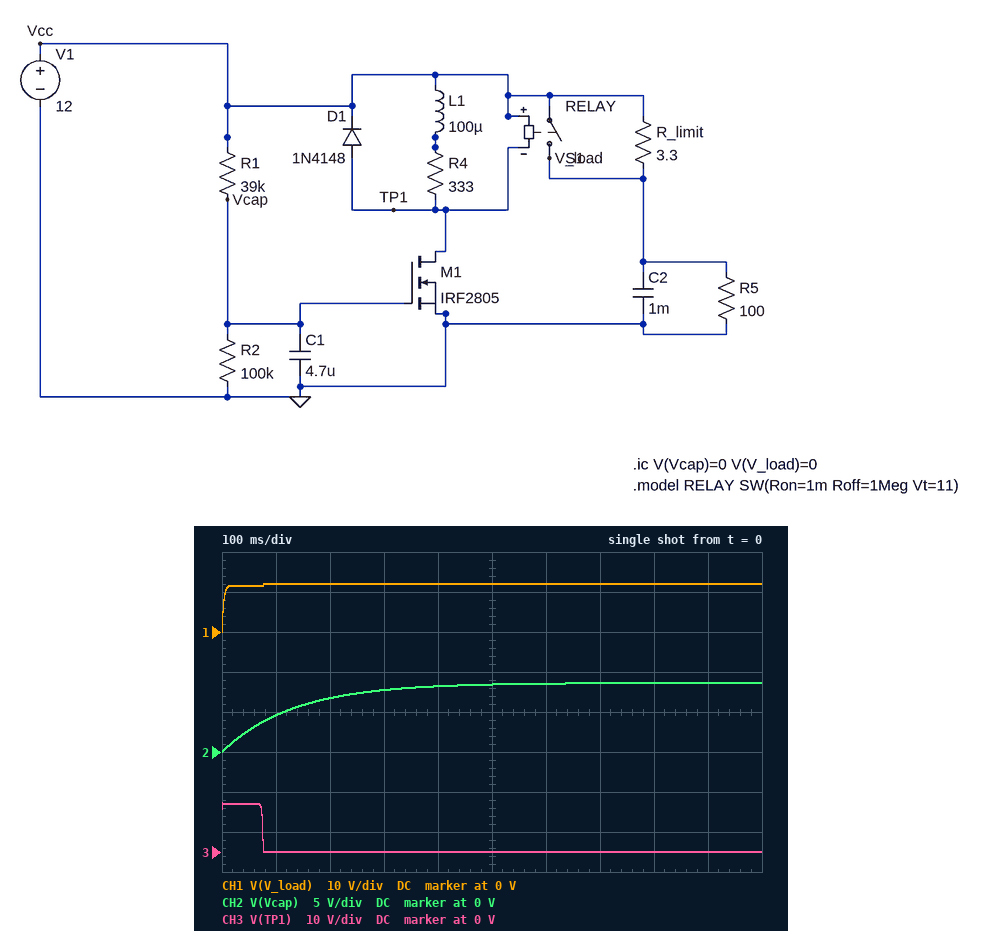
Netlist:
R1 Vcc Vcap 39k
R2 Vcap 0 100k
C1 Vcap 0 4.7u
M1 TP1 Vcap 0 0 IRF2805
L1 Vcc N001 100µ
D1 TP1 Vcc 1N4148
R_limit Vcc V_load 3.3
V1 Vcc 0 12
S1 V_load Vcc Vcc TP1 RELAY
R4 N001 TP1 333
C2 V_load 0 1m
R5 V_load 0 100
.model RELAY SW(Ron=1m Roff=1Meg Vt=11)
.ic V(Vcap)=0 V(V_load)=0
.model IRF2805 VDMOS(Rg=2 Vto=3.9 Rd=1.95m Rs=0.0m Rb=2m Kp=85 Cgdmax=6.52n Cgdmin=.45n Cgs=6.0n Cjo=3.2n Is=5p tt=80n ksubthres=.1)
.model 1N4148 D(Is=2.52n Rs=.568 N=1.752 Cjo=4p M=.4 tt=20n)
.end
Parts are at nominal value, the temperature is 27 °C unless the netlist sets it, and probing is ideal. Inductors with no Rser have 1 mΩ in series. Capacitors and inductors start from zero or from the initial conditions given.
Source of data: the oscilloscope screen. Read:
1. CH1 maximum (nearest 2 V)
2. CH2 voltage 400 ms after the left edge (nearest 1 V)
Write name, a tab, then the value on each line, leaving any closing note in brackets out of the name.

CH1 maximum	12 V
CH2 voltage 400 ms after the left edge	8 V
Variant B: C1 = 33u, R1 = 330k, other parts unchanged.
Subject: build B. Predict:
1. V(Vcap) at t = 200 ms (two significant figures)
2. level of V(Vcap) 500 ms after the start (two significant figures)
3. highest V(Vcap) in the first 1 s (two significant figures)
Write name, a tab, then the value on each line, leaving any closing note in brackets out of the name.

V(Vcap) at t = 200 ms	210 mV
level of V(Vcap) 500 ms after the start	500 mV
highest V(Vcap) in the first 1 s	910 mV
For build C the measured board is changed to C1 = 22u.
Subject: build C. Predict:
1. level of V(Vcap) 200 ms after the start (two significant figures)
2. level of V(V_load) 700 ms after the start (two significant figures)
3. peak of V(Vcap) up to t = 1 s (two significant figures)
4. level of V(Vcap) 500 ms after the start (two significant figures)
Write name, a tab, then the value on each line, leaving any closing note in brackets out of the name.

level of V(Vcap) 200 ms after the start	2.4 V
level of V(V_load) 700 ms after the start	12 V
peak of V(Vcap) up to t = 1 s	6.9 V
level of V(Vcap) 500 ms after the start	4.8 V
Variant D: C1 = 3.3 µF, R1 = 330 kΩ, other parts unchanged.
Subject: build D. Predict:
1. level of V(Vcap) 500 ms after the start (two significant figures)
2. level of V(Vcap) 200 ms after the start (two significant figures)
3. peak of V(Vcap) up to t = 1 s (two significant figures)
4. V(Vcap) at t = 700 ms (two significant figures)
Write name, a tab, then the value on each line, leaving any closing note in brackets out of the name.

level of V(Vcap) 500 ms after the start	2.4 V
level of V(Vcap) 200 ms after the start	1.5 V
peak of V(Vcap) up to t = 1 s	2.7 V
V(Vcap) at t = 700 ms	2.6 V
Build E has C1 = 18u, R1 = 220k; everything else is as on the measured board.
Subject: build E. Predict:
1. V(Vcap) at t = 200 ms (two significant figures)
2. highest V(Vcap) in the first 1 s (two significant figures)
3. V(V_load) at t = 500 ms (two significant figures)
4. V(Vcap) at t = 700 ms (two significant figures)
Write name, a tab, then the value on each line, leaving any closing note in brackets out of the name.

V(Vcap) at t = 200 ms	560 mV
highest V(Vcap) in the first 1 s	2.1 V
V(V_load) at t = 500 ms	12 V
V(Vcap) at t = 700 ms	1.6 V
